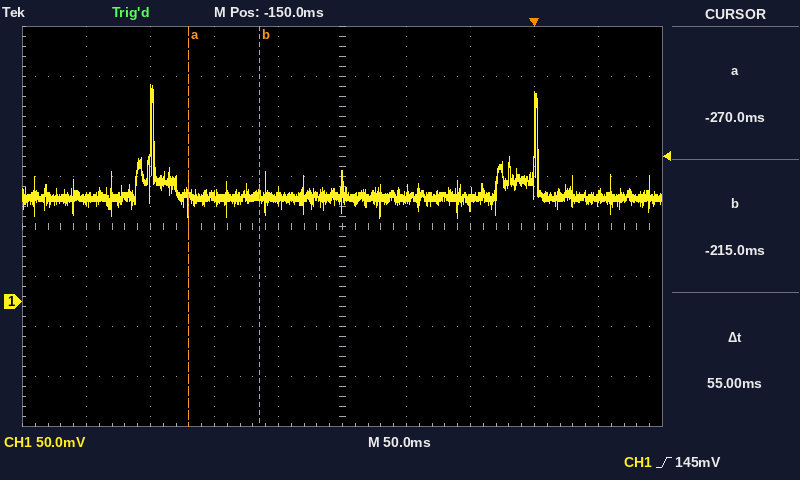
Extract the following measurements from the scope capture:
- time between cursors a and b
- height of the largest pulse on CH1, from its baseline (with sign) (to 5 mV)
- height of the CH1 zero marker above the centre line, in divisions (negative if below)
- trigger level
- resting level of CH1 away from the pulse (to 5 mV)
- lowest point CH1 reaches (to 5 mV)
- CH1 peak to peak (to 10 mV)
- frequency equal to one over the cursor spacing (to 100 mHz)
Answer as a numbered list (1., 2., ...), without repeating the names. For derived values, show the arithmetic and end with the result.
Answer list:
1. 55 ms
2. +115 mV
3. -1.5 div
4. 145 mV
5. 105 mV
6. 85 mV
7. 130 mV
8. 1 / 55 ms ≈ 18.2 Hz
